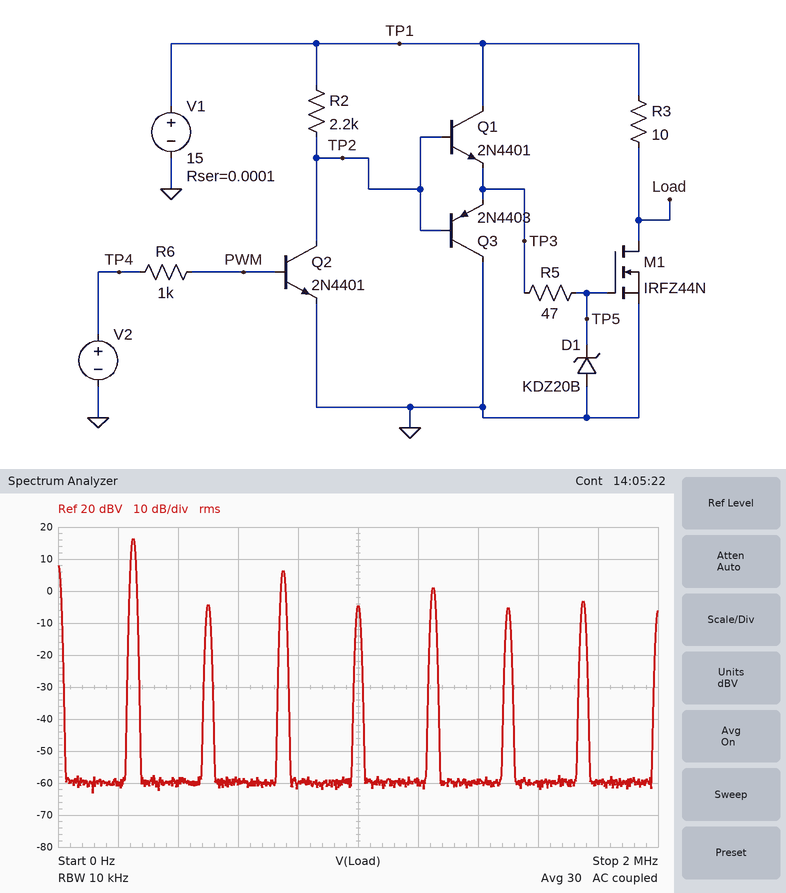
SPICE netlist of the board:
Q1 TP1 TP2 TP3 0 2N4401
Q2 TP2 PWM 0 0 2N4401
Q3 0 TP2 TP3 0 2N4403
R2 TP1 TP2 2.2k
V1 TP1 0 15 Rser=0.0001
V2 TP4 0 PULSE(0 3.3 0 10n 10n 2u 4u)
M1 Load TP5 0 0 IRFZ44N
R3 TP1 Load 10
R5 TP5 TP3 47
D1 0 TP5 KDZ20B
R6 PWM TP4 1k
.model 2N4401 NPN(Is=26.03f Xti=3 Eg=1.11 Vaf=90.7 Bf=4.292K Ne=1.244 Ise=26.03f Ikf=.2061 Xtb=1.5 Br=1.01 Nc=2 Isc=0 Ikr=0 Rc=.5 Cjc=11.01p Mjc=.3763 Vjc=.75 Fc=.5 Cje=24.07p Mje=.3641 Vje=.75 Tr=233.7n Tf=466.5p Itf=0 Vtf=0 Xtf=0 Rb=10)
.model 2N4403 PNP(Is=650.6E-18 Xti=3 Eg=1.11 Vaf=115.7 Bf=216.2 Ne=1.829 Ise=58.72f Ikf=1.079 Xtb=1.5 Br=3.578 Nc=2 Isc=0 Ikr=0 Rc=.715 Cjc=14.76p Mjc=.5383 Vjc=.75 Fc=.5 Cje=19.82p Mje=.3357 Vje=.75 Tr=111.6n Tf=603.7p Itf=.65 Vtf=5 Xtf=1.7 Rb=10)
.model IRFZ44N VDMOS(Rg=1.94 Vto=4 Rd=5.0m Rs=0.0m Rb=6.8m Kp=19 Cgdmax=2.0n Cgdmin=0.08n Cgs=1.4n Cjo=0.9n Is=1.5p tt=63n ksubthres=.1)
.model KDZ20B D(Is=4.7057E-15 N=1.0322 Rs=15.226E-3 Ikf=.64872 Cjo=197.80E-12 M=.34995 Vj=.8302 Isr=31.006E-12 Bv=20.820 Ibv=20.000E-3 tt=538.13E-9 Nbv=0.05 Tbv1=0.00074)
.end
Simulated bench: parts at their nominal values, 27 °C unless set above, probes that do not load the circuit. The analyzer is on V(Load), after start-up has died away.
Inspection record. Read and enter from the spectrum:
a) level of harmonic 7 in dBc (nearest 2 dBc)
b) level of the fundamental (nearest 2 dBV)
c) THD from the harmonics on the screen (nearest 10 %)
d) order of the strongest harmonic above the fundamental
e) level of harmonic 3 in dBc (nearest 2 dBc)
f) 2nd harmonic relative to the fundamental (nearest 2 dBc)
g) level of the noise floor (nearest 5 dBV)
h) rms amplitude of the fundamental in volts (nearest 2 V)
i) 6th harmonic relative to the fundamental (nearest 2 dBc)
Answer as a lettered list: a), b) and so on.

a) -20 dBc
b) 16 dBV
c) 40 %
d) 3
e) -10 dBc
f) -20 dBc
g) -60 dBV
h) 6 V
i) -22 dBc
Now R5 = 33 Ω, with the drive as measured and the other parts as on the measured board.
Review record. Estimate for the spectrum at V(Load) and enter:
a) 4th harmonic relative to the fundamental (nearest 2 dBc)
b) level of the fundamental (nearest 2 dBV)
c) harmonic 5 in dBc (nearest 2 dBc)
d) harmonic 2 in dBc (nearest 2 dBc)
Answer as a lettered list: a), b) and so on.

a) -16 dBc
b) 16 dBV
c) -18 dBc
d) -16 dBc
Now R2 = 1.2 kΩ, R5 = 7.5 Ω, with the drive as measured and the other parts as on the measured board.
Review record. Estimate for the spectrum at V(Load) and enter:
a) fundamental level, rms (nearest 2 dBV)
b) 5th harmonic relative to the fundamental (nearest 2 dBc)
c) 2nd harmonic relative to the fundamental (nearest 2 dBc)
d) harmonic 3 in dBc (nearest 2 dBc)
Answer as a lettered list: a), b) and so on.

a) 16 dBV
b) -26 dBc
c) -12 dBc
d) -12 dBc
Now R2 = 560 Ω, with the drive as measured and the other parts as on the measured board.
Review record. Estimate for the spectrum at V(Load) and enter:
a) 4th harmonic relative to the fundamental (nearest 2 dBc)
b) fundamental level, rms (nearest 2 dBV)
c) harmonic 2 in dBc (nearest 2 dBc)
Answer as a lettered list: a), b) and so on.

a) -26 dBc
b) 16 dBV
c) -26 dBc
